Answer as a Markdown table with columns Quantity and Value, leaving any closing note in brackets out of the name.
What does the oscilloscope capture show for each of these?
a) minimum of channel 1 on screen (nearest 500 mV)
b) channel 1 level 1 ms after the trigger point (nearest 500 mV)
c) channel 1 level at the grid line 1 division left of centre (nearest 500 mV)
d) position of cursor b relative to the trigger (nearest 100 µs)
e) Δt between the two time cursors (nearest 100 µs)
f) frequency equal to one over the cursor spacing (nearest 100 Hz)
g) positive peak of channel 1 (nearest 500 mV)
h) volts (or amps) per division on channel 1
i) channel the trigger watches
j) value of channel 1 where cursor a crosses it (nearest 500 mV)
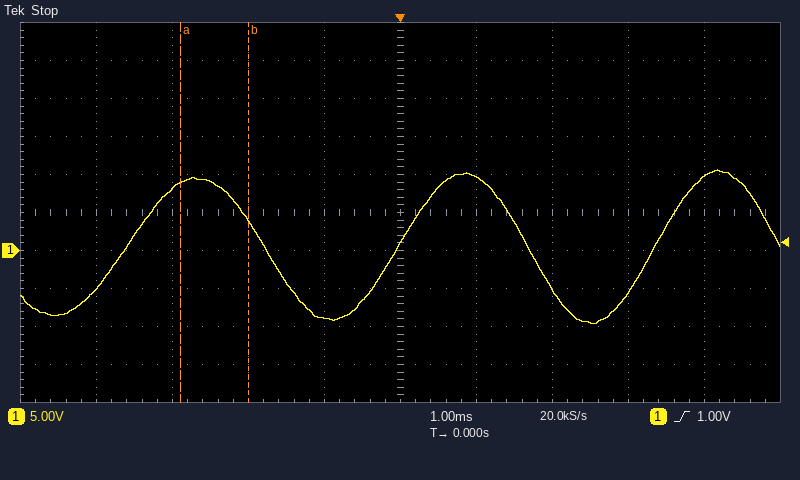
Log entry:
| Quantity | Value |
|---|---|
| minimum of channel 1 on screen | -9.5 V |
| channel 1 level 1 ms after the trigger point | 9.5 V |
| channel 1 level at the grid line 1 division left of centre | -9.0 V |
| position of cursor b relative to the trigger | -2.0 ms |
| Δt between the two time cursors | 900 µs |
| frequency equal to one over the cursor spacing | 1.1 kHz |
| positive peak of channel 1 | 10.5 V |
| volts (or amps) per division on channel 1 | 5 V |
| channel the trigger watches | channel 1 |
| value of channel 1 where cursor a crosses it | 9.0 V |
